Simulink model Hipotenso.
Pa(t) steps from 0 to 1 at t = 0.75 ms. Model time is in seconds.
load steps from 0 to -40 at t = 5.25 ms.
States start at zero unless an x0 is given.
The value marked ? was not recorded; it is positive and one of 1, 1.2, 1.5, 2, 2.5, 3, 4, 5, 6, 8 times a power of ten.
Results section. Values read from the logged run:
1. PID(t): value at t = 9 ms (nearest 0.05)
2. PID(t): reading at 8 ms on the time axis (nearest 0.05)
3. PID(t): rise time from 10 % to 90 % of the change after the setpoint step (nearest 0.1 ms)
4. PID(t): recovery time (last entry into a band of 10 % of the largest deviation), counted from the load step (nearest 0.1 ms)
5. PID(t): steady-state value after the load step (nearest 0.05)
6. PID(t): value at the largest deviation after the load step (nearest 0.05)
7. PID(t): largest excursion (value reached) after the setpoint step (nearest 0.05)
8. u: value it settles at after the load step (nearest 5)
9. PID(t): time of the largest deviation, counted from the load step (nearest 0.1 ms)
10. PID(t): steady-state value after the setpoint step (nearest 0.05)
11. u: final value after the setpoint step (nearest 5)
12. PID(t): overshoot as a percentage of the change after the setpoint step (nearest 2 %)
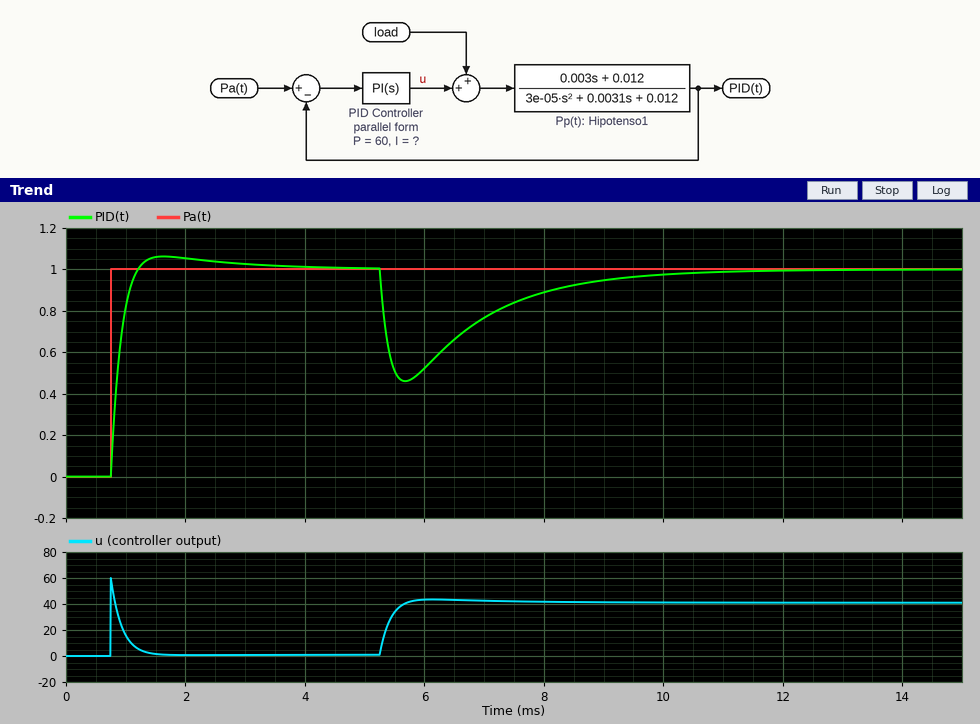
0.95
0.90
0.3 ms
3.7 ms
1.00
0.45
1.05
40
0.4 ms
1.00
0
6 %
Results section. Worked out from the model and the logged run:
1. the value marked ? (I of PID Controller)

40000
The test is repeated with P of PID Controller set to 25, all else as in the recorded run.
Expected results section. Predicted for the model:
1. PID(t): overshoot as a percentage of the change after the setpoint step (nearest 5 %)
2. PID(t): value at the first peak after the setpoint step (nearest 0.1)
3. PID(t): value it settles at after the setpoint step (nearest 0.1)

20 %
1.2
1.0
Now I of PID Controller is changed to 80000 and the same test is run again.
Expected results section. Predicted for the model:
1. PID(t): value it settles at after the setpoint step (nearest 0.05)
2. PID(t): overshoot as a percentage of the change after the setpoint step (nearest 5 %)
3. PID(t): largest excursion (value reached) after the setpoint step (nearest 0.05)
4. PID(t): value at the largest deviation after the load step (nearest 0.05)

1.00
10 %
1.10
0.50
